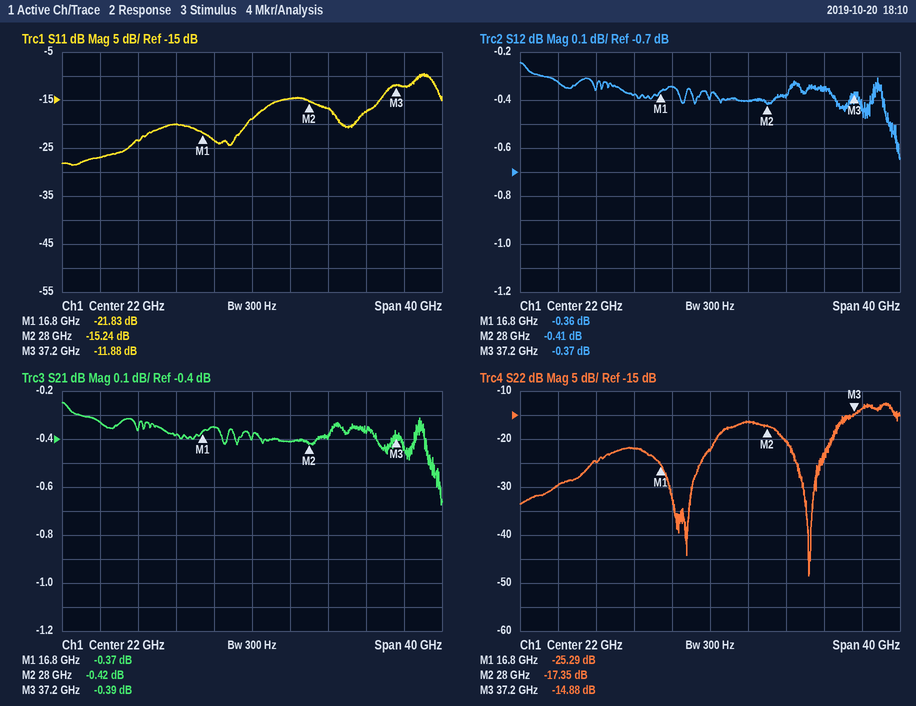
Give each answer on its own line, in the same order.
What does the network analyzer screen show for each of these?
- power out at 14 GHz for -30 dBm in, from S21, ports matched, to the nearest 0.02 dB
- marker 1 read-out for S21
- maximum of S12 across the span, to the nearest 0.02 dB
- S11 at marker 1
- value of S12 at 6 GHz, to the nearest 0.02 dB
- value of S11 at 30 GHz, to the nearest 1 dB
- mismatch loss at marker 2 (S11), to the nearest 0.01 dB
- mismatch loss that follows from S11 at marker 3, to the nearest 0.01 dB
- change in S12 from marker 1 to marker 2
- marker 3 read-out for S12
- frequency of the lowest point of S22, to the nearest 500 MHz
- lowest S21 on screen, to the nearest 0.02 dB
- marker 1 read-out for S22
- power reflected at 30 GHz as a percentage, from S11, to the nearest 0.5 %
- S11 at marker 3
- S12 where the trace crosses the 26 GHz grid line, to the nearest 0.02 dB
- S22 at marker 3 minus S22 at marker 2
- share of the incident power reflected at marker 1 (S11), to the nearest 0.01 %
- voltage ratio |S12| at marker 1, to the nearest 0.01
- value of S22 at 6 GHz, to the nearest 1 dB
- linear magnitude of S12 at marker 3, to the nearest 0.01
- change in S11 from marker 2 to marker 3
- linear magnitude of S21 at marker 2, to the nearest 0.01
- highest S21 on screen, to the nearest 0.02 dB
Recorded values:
-30.38 dBm
-0.37 dB
-0.24 dB
-21.83 dB
-0.32 dB
-17 dB
0.13 dB
0.29 dB
-0.05 dB
-0.37 dB
32.5 GHz
-0.68 dB
-25.29 dB
2.0 %
-11.88 dB
-0.40 dB
2.47 dB
0.66 %
0.96
-30 dB
0.96
3.36 dB
0.95
-0.24 dB
